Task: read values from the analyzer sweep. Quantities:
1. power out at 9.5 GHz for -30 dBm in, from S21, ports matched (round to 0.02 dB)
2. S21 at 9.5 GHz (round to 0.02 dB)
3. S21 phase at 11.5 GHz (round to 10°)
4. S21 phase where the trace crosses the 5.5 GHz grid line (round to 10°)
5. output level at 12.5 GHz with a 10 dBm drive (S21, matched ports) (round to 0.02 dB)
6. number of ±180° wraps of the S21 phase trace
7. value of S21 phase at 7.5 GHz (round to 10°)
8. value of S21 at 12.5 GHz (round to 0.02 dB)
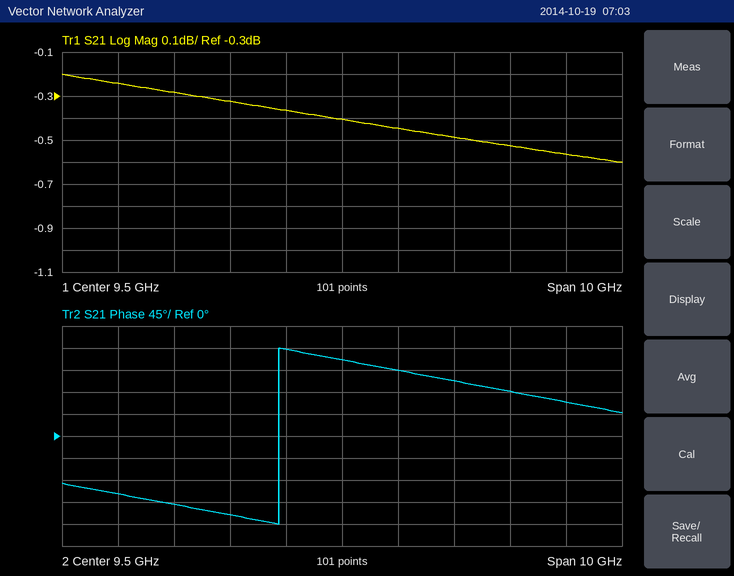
-30.40 dBm
-0.40 dB
110°
-120°
9.48 dBm
1
-160°
-0.52 dB
